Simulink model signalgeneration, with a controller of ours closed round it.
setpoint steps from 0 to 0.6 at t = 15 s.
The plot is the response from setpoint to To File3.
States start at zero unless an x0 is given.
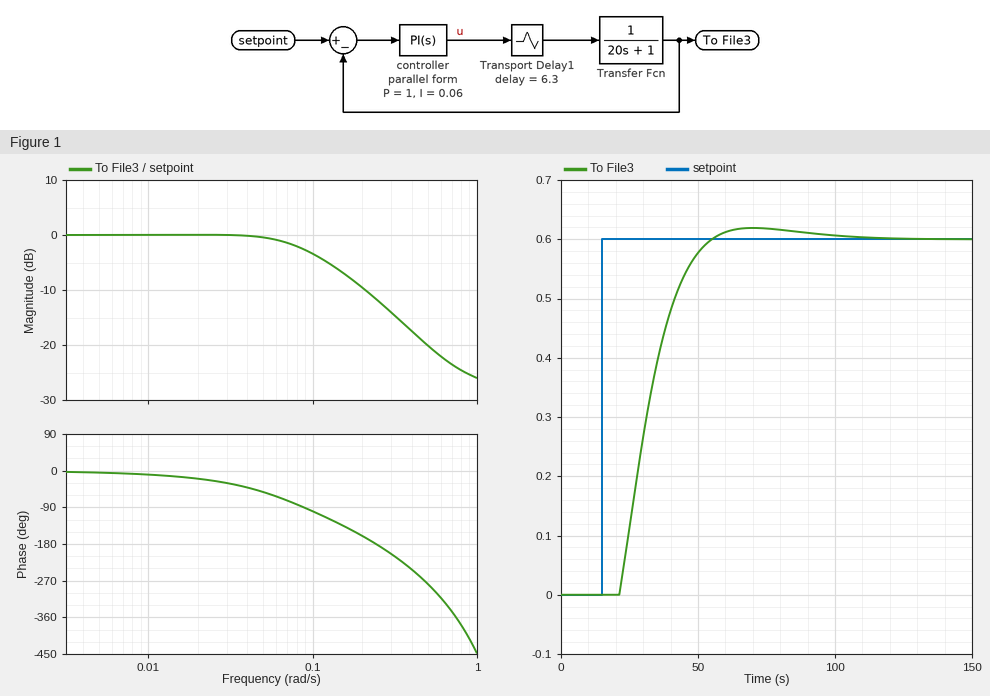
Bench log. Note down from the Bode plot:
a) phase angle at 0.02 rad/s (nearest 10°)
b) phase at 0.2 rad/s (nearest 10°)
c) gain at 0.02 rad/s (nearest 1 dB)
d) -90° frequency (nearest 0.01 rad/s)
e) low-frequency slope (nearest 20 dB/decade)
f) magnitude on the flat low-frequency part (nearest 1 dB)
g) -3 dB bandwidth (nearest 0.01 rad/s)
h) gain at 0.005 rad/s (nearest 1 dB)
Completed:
-20°
-160°
0 dB
0.09 rad/s
0 dB/decade
0 dB
0.09 rad/s
0 dB
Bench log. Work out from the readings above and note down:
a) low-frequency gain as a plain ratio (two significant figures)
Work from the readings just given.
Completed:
1.0
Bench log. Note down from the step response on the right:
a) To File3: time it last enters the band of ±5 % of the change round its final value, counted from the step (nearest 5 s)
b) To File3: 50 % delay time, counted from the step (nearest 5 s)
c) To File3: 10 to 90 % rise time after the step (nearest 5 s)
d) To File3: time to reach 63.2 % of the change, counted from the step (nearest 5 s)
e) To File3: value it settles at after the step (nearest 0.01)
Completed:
35 s
15 s
20 s
20 s
0.60
